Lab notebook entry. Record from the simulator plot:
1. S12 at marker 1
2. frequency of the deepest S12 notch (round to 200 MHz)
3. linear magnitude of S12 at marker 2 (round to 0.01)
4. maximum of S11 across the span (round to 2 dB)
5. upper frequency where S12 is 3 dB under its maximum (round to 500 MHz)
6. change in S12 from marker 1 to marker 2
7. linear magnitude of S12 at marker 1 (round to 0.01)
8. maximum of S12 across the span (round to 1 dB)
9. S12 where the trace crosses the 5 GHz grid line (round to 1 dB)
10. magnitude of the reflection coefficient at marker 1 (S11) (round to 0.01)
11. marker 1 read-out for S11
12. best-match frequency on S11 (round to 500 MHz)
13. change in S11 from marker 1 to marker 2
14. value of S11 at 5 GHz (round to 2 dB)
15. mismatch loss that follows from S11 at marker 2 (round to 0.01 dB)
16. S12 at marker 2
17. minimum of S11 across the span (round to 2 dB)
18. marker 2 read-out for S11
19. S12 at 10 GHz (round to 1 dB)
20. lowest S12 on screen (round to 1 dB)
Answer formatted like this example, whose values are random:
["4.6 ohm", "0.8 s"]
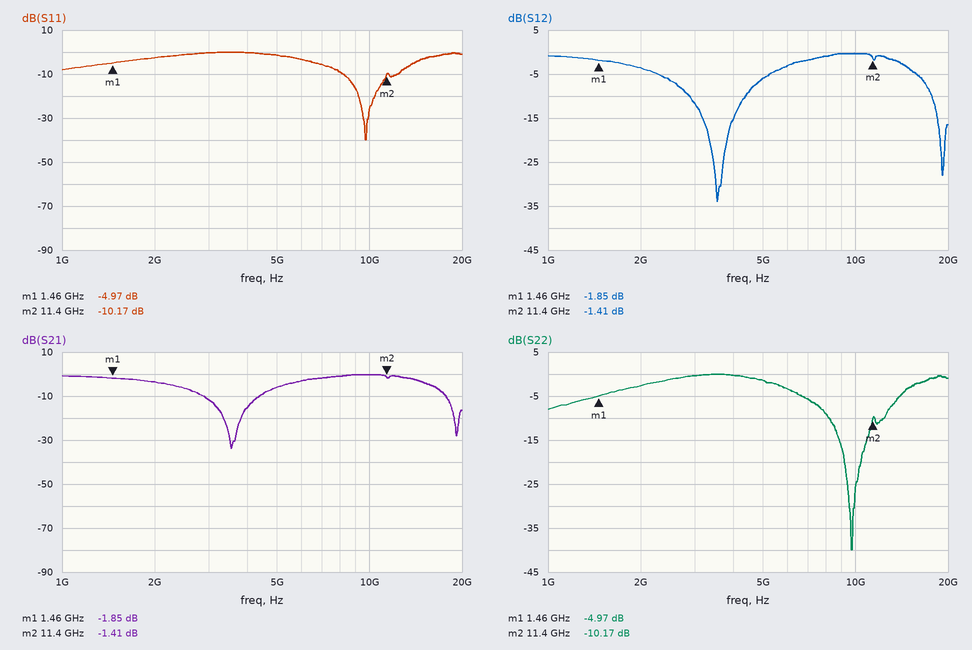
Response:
["-1.85 dB", "3.6 GHz", "0.85", "0 dB", "14.5 GHz", "0.44 dB", "0.81", "0 dB", "-6 dB", "0.56", "-4.97 dB", "9.5 GHz", "-5.20 dB", "-2 dB", "0.44 dB", "-1.41 dB", "-40 dB", "-10.17 dB", "0 dB", "-34 dB"]
